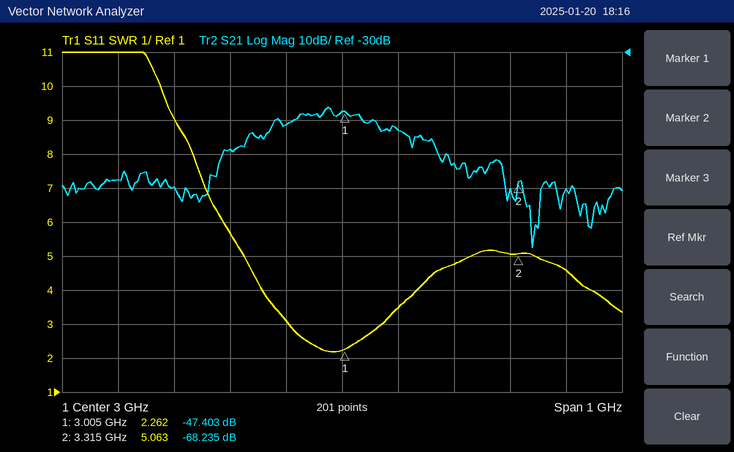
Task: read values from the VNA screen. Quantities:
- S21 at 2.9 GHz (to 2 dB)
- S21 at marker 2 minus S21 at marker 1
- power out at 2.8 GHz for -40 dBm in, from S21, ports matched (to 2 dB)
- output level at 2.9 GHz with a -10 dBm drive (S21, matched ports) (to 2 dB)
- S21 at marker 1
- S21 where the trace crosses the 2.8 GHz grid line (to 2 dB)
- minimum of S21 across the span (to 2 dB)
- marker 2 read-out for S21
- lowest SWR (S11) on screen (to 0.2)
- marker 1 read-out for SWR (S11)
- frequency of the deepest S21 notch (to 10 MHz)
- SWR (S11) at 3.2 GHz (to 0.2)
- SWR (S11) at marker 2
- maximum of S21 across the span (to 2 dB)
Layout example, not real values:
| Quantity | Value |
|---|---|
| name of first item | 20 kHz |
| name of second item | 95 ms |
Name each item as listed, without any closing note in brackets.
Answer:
| Quantity | Value |
|---|---|
| S21 at 2.9 GHz | -52 dB |
| S21 at marker 2 minus S21 at marker 1 | -20.832 dB |
| power out at 2.8 GHz for -40 dBm in, from S21, ports matched | -98 dBm |
| output level at 2.9 GHz with a -10 dBm drive (S21, matched ports) | -62 dBm |
| S21 at marker 1 | -47.403 dB |
| S21 where the trace crosses the 2.8 GHz grid line | -58 dB |
| minimum of S21 across the span | -88 dB |
| marker 2 read-out for S21 | -68.235 dB |
| lowest SWR (S11) on screen | 2.2 |
| marker 1 read-out for SWR | 2.262 |
| frequency of the deepest S21 notch | 3.34 GHz |
| SWR (S11) at 3.2 GHz | 4.8 |
| SWR (S11) at marker 2 | 5.063 |
| maximum of S21 across the span | -46 dB |
